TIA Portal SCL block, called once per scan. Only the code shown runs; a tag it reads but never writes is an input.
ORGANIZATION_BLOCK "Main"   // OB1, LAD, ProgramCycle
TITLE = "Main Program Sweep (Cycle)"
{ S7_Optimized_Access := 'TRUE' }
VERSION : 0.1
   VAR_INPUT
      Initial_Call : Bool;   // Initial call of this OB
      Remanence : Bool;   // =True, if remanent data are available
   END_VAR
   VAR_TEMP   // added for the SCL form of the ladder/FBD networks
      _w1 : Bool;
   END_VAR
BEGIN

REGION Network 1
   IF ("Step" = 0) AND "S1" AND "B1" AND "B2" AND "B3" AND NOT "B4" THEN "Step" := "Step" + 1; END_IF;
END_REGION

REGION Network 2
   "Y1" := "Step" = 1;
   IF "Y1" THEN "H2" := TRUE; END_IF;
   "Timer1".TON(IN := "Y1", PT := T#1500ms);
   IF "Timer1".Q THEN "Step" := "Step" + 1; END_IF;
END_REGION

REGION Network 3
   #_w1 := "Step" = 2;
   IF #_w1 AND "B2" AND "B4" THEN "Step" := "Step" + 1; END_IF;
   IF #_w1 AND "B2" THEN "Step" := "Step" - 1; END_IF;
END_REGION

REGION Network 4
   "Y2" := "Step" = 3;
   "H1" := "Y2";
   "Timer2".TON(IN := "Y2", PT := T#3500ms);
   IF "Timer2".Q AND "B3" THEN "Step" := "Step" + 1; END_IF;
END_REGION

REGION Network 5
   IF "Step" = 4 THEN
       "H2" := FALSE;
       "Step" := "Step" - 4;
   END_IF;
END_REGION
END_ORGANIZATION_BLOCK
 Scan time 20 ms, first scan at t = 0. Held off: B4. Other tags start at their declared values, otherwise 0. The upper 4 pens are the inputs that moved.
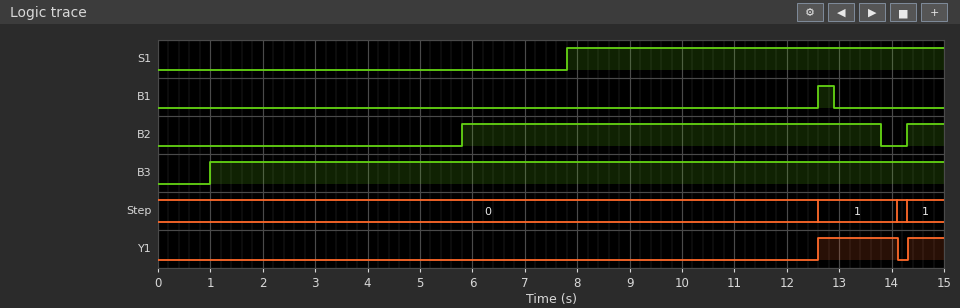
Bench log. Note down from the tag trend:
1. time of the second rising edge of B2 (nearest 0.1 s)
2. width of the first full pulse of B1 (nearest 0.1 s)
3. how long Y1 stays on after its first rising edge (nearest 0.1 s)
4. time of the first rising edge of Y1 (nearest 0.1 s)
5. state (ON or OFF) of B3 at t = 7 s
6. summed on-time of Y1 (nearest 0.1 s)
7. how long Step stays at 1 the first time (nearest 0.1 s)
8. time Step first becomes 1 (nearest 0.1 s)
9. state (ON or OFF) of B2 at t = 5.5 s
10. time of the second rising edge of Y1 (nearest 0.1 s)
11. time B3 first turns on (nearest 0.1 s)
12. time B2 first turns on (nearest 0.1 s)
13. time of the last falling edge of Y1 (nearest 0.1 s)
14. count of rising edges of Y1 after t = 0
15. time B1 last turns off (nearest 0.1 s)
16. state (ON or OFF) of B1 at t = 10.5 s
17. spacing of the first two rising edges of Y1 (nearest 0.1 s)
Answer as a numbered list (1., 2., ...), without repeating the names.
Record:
1. 14.3 s
2. 0.3 s
3. 1.5 s
4. 12.6 s
5. ON
6. 2.2 s
7. 1.5 s
8. 12.6 s
9. OFF
10. 14.3 s
11. 1.0 s
12. 5.8 s
13. 14.1 s
14. 2
15. 12.9 s
16. OFF
17. 1.7 s
